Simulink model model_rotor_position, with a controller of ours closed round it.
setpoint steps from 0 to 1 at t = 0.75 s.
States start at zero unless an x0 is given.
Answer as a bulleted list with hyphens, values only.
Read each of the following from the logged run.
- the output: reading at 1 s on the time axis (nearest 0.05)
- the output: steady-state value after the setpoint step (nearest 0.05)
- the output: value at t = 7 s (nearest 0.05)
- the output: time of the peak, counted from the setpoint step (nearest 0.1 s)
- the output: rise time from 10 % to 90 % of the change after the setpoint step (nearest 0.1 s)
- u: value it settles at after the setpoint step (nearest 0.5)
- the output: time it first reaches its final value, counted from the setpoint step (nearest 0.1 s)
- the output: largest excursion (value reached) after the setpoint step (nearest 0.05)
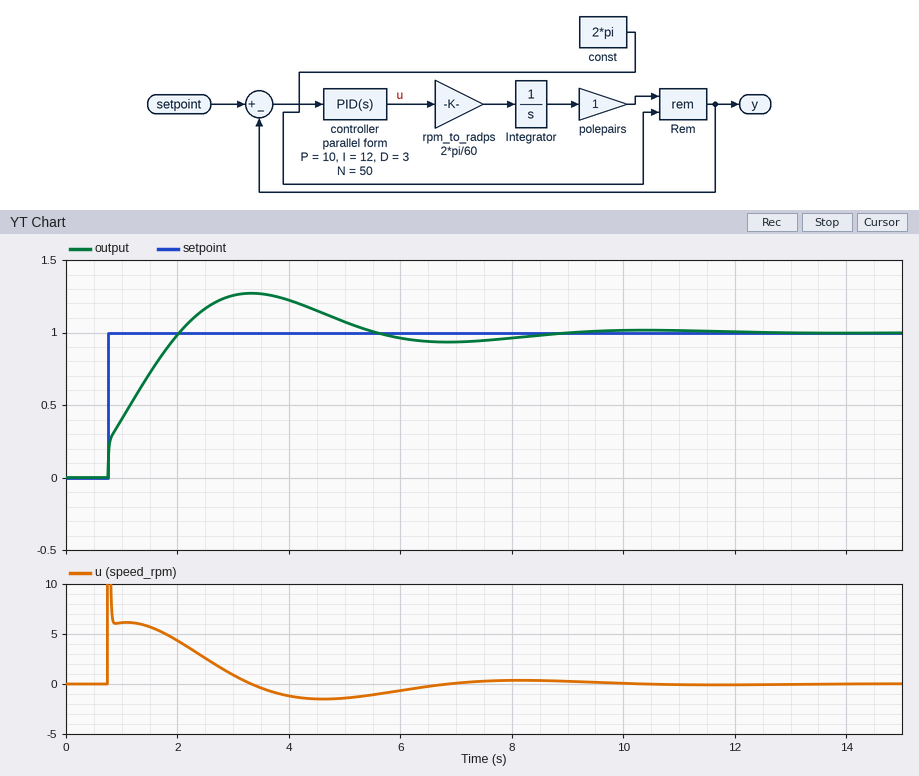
- 0.40
- 1.00
- 0.95
- 2.6 s
- 1.1 s
- 0.0
- 1.3 s
- 1.25
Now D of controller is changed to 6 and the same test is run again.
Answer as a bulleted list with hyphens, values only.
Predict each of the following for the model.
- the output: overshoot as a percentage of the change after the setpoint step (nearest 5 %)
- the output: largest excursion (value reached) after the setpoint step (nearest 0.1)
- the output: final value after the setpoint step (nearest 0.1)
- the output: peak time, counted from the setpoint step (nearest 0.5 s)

- 25 %
- 1.2
- 1.0
- 3.0 s
